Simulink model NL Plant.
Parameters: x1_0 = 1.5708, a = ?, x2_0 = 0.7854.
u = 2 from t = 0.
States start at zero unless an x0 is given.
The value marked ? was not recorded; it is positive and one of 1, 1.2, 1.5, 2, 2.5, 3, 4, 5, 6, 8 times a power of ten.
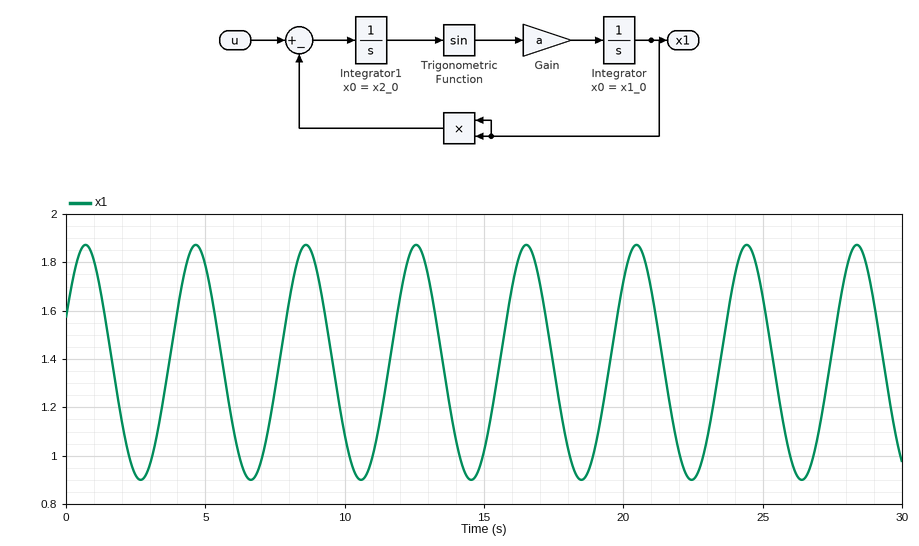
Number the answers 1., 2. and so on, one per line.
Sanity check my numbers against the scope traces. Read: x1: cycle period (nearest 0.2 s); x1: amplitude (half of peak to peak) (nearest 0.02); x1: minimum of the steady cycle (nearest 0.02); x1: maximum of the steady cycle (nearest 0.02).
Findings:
1. 4.0 s
2. 0.48
3. 0.90
4. 1.88
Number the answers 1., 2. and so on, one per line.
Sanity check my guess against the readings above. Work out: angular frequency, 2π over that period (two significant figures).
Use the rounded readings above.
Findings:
1. 1.6 rad/s
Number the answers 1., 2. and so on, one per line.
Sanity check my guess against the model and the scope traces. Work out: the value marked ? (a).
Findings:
1. 1
